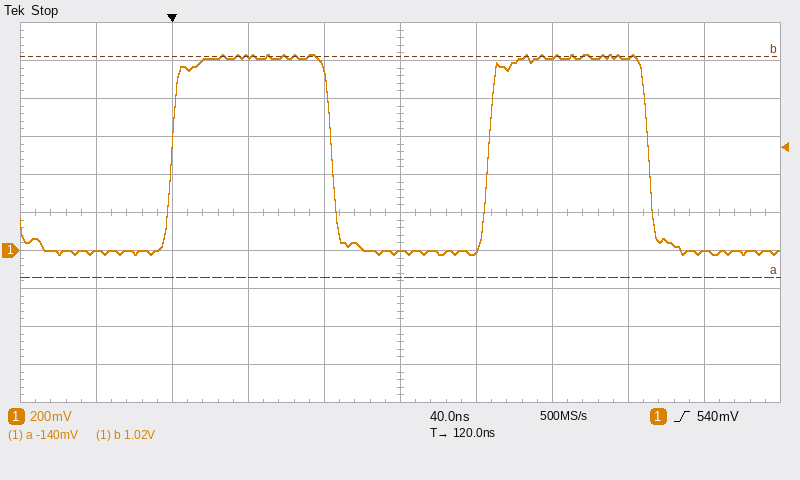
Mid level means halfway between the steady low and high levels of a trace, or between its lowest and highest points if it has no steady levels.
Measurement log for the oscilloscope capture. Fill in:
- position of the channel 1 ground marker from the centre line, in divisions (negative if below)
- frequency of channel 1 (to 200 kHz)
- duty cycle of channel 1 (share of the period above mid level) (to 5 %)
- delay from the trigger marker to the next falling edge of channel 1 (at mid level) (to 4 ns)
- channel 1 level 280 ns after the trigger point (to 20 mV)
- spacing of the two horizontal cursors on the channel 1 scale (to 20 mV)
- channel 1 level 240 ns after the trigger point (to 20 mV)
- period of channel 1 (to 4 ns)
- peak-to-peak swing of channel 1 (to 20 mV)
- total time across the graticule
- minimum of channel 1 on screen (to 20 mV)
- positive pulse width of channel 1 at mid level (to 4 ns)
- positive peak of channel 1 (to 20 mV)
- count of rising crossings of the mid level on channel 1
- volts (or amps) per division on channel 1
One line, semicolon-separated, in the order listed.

-1.0 div; 6.0 MHz; 50 %; 84 ns; 0 mV; 1.16 V; 1.02 V; 168 ns; 1.06 V; 400 ns; -20 mV; 84 ns; 1.04 V; 2; 200 mV
